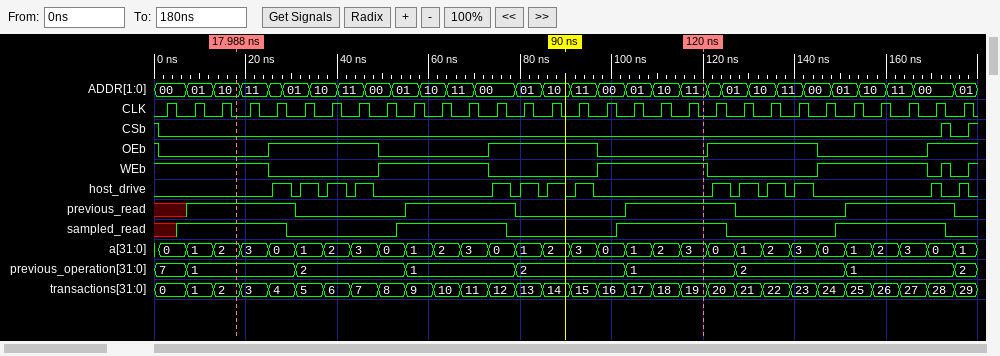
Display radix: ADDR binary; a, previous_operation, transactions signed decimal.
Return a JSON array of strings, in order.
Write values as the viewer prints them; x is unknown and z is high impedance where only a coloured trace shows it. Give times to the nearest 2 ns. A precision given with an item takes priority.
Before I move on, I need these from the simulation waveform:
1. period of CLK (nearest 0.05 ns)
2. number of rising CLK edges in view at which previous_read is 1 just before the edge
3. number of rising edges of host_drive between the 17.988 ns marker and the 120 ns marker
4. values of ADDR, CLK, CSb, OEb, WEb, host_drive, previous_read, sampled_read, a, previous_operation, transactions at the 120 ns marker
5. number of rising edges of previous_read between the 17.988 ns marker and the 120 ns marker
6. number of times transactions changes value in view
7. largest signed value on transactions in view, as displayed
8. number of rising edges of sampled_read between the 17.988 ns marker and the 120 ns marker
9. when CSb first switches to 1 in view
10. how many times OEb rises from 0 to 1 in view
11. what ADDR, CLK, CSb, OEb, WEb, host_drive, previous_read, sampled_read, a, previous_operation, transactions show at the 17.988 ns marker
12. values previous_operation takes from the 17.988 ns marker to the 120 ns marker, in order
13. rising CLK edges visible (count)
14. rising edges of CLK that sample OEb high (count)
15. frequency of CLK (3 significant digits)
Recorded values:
["6 ns", "16", "8", "ADDR=11, CLK=0, CSb=0, OEb=0, WEb=1, host_drive=0, previous_read=1, sampled_read=1, a=3, previous_operation=1, transactions=19", "2", "29", "29", "2", "172 ns", "4", "ADDR=10, CLK=0, CSb=0, OEb=0, WEb=1, host_drive=0, previous_read=1, sampled_read=1, a=2, previous_operation=1, transactions=2", "1, 2, 1, 2, 1", "30", "14", "167 MHz"]
